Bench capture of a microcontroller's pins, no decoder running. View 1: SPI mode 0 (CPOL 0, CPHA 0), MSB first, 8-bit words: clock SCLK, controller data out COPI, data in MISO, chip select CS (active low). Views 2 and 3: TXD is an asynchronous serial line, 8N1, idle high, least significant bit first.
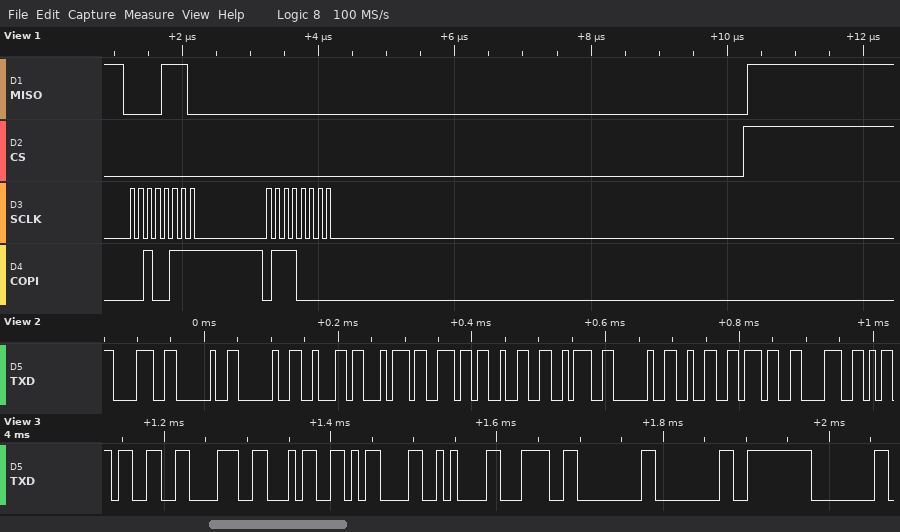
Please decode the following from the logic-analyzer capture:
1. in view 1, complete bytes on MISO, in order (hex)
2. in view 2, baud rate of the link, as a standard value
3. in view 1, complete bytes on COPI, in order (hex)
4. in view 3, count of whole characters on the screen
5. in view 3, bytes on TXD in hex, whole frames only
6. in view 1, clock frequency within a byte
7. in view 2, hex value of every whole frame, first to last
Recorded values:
0x0E 0x00
115200 baud
0x27 0x70
10
33 38 34 0D 0A 3C 00 00 FE 00
8 MHz
0x38 0x20 0x20 0x62 0x74 0x6E 0x32 0x3A 0x20 0x32 0x37 0x38
